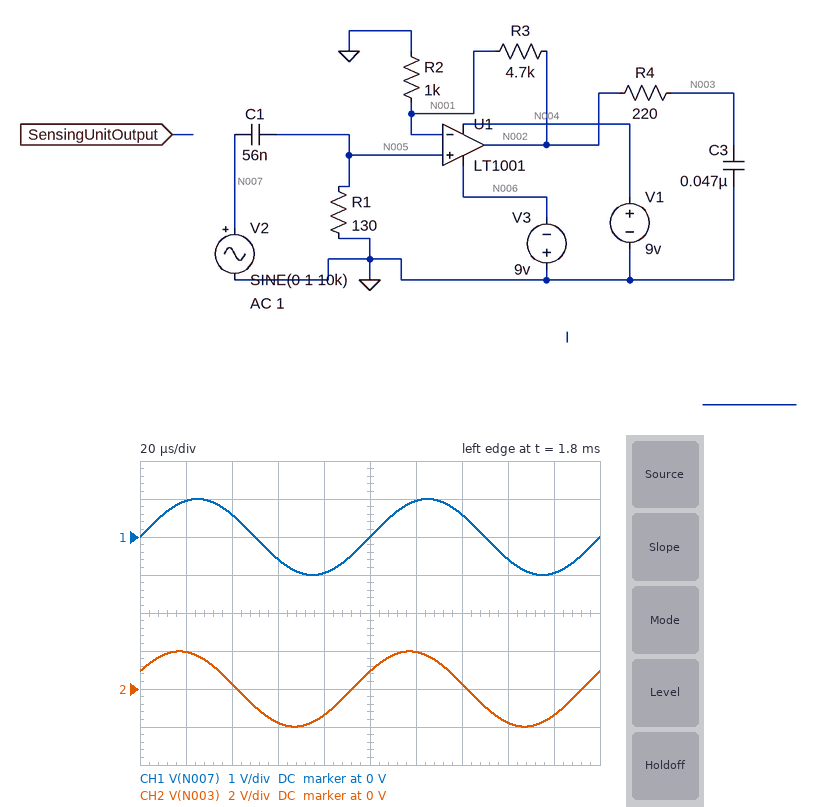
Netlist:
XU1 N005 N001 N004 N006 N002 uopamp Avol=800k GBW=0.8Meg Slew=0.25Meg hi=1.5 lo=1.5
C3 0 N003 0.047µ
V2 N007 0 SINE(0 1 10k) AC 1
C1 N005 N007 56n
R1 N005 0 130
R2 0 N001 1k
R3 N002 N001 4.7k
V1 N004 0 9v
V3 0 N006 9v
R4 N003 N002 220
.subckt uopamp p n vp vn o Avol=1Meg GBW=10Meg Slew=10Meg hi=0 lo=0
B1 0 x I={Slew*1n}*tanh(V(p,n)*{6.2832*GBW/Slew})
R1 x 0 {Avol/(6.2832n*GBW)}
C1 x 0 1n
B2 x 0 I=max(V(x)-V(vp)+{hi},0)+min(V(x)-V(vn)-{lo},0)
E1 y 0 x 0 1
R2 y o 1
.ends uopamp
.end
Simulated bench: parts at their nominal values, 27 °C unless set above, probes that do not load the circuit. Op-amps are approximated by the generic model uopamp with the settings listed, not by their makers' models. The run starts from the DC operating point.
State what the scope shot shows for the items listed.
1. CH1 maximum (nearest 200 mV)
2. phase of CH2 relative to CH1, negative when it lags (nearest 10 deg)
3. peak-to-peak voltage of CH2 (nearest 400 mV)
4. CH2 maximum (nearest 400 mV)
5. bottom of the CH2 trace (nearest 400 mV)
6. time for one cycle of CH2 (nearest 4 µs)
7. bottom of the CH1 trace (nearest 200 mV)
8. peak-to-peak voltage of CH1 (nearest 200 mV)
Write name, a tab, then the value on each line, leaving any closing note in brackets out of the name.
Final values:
CH1 maximum	1.0 V
phase of CH2 relative to CH1, negative when it lags	30 deg
peak-to-peak voltage of CH2	4.0 V
CH2 maximum	2.0 V
bottom of the CH2 trace	-2.0 V
time for one cycle of CH2	100 µs
bottom of the CH1 trace	-1.0 V
peak-to-peak voltage of CH1	2.0 V
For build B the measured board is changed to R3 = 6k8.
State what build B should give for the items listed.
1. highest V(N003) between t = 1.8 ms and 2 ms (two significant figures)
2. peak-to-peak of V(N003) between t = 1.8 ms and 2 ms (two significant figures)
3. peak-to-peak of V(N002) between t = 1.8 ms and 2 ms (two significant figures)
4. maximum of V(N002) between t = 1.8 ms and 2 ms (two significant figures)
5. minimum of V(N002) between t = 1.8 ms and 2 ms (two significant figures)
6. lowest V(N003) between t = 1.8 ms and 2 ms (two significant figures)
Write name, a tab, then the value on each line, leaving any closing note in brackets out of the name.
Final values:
highest V(N003) between t = 1.8 ms and 2 ms	2.7 V
peak-to-peak of V(N003) between t = 1.8 ms and 2 ms	5.4 V
peak-to-peak of V(N002) between t = 1.8 ms and 2 ms	6.5 V
maximum of V(N002) between t = 1.8 ms and 2 ms	3.2 V
minimum of V(N002) between t = 1.8 ms and 2 ms	-3.2 V
lowest V(N003) between t = 1.8 ms and 2 ms	-2.7 V
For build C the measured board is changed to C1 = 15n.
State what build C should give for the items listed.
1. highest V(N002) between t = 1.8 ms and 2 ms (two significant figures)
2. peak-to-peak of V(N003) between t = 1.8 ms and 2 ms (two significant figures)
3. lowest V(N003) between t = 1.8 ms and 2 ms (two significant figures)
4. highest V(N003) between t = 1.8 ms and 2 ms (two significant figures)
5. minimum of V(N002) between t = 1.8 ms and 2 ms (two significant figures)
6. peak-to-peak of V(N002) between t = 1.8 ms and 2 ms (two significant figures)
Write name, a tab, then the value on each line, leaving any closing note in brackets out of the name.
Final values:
highest V(N002) between t = 1.8 ms and 2 ms	690 mV
peak-to-peak of V(N003) between t = 1.8 ms and 2 ms	1.2 V
lowest V(N003) between t = 1.8 ms and 2 ms	-580 mV
highest V(N003) between t = 1.8 ms and 2 ms	580 mV
minimum of V(N002) between t = 1.8 ms and 2 ms	-690 mV
peak-to-peak of V(N002) between t = 1.8 ms and 2 ms	1.4 V
